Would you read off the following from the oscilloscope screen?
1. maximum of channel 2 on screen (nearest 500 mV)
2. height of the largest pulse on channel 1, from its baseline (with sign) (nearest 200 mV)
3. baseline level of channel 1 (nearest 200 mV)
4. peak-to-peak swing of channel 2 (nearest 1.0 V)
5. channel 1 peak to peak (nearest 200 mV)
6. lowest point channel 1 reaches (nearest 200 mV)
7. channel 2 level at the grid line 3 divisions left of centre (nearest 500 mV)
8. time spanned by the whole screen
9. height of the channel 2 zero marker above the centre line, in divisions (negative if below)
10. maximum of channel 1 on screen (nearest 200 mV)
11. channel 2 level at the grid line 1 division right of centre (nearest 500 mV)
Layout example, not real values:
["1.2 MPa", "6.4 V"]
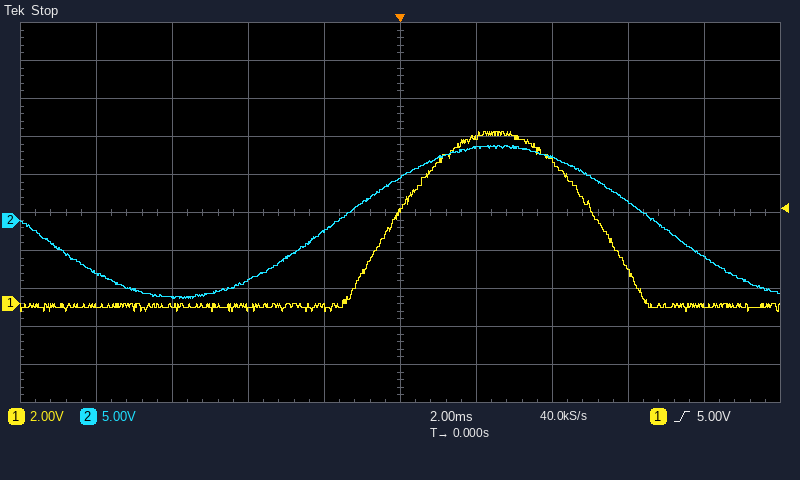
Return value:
["10.0 V", "+9.2 V", "-200 mV", "20.0 V", "9.4 V", "-400 mV", "-10.0 V", "20 ms", "-0.2 div", "9.0 V", "9.5 V"]
